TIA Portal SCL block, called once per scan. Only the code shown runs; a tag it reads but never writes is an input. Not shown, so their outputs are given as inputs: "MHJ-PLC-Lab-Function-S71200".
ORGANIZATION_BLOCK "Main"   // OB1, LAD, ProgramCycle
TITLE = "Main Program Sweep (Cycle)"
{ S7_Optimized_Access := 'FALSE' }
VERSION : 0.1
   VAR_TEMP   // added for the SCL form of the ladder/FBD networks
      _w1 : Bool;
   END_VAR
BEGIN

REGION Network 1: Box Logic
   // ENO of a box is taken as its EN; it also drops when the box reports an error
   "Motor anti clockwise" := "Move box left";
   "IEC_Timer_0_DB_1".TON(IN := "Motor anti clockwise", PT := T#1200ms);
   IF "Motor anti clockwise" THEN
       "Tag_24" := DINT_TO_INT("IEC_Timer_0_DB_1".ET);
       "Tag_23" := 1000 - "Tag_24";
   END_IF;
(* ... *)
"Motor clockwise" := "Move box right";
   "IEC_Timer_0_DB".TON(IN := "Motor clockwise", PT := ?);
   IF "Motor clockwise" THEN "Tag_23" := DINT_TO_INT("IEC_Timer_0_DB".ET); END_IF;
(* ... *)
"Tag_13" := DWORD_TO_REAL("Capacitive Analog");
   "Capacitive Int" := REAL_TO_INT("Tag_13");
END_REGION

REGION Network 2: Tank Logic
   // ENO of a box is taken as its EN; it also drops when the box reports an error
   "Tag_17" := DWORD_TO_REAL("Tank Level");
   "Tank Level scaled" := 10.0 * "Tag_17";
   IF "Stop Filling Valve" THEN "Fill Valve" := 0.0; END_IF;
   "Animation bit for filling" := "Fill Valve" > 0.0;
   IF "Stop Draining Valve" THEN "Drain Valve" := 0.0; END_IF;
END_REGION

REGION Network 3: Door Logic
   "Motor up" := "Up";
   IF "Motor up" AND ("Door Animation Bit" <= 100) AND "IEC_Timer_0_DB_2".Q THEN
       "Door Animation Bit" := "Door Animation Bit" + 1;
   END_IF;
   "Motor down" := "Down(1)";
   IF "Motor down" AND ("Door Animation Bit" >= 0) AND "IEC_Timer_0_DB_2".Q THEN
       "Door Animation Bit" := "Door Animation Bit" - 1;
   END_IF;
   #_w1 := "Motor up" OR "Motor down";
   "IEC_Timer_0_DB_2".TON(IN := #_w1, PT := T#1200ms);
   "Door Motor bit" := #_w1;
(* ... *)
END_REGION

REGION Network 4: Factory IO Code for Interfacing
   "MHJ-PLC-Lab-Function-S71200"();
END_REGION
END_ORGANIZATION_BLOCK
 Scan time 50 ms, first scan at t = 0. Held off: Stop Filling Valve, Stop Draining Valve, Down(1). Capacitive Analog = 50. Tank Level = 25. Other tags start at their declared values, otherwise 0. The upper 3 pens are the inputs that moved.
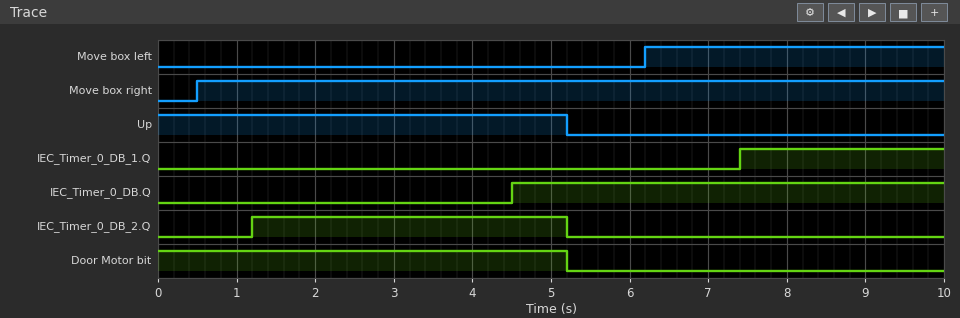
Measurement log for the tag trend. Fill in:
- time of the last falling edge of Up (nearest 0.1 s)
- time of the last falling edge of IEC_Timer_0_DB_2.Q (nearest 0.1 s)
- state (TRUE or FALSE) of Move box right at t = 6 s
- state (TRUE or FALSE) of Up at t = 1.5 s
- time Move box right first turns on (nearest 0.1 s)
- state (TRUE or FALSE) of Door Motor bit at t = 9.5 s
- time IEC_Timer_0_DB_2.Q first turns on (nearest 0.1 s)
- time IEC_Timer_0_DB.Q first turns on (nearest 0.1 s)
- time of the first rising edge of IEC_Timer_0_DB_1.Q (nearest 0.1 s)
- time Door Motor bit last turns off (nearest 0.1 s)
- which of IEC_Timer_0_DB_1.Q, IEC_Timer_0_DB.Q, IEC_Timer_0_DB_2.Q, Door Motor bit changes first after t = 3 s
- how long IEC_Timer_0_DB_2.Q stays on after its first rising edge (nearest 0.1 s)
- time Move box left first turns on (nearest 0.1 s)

5.2 s
5.2 s
TRUE
TRUE
0.5 s
FALSE
1.2 s
4.5 s
7.4 s
5.2 s
IEC_Timer_0_DB.Q
4.0 s
6.2 s
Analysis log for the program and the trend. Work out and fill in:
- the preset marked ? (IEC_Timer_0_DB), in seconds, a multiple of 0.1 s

4.0 s
